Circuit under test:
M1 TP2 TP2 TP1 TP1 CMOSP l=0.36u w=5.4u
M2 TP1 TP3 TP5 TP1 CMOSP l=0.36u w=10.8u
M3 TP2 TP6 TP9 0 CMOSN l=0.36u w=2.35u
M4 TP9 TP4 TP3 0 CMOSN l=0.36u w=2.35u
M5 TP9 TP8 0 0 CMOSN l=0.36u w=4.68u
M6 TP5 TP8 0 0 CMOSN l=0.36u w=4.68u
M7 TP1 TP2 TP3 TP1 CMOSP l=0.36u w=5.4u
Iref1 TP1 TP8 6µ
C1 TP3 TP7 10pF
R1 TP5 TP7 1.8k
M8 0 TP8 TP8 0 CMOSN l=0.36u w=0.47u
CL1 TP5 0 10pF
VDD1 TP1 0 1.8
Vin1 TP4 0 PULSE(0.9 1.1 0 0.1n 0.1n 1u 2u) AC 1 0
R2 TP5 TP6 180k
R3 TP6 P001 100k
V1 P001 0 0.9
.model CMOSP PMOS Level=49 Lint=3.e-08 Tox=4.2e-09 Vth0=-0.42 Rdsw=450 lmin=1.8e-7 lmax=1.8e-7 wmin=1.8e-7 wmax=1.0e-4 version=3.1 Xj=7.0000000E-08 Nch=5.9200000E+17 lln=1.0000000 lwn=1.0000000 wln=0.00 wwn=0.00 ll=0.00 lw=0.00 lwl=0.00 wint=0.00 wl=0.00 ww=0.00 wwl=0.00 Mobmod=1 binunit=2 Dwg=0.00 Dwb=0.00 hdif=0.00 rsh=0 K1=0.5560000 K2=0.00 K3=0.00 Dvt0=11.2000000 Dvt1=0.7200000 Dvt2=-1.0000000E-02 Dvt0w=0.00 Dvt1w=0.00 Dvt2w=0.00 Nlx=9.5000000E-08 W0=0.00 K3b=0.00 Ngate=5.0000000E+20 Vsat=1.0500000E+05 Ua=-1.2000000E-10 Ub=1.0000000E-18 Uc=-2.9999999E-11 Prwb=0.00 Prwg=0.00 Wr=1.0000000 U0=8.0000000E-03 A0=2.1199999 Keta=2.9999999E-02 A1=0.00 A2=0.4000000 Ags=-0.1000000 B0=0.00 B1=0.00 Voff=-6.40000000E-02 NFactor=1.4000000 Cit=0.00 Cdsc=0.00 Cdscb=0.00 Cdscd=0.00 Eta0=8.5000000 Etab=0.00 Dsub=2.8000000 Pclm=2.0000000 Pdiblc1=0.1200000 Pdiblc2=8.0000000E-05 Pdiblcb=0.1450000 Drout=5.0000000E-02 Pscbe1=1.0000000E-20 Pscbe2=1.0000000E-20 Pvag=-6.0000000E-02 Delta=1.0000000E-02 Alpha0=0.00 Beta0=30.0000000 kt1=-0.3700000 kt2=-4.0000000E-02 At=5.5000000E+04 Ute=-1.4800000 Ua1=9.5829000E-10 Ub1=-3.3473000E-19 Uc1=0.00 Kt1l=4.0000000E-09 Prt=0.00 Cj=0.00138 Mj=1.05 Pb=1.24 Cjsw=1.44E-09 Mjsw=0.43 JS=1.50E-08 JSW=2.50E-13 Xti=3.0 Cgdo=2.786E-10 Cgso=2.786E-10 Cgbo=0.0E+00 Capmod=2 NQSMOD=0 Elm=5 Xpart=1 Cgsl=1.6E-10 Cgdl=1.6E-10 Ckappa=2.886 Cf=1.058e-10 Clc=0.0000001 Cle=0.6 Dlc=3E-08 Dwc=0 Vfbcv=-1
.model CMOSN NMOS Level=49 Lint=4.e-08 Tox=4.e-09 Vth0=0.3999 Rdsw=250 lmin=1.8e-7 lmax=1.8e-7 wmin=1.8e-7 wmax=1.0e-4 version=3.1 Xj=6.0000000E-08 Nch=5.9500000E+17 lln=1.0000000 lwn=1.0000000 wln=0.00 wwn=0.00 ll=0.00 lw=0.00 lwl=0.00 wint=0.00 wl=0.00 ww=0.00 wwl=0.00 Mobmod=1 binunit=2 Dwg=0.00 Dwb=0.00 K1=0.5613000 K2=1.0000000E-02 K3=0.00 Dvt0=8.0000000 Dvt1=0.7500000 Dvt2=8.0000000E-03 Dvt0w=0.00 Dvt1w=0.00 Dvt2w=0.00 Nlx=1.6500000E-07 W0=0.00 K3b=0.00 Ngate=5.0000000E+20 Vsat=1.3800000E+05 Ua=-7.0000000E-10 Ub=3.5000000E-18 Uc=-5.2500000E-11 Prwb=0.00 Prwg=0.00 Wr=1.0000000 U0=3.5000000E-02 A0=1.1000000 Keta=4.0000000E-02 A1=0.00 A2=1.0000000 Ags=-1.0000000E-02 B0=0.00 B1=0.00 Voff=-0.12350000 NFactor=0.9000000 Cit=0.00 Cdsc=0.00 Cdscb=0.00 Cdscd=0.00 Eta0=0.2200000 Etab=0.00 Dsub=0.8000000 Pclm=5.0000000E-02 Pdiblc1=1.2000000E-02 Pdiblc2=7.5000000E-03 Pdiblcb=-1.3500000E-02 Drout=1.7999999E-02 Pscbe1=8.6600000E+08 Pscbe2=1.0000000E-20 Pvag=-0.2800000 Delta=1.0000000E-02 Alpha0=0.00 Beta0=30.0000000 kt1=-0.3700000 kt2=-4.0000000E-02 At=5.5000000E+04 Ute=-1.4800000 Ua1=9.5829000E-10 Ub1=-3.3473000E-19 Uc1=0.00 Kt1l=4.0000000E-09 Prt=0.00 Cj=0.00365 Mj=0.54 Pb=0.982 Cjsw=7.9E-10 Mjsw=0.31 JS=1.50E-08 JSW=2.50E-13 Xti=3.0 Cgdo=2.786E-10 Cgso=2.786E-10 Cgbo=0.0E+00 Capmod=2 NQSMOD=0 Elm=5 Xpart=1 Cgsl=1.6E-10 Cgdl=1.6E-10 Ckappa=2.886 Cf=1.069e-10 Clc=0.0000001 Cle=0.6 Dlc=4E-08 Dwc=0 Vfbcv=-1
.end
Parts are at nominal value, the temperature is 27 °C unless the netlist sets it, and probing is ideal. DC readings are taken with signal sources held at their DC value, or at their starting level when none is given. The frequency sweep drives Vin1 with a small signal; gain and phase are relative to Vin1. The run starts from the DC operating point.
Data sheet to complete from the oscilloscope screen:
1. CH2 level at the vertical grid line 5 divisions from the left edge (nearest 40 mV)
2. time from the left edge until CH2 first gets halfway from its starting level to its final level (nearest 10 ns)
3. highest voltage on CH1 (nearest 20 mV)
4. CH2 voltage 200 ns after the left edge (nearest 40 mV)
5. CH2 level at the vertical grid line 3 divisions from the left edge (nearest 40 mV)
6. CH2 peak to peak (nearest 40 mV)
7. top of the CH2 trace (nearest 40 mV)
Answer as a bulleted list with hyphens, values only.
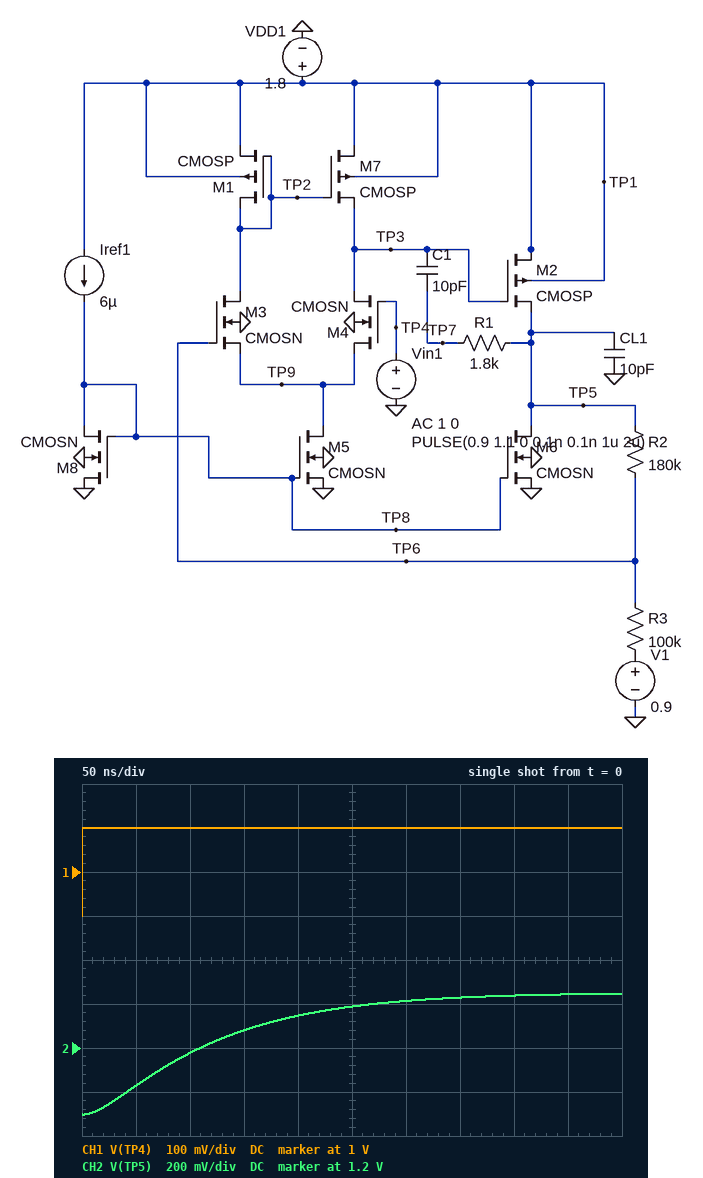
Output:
- 1.40 V
- 100 ns
- 1.10 V
- 1.36 V
- 1.28 V
- 560 mV
- 1.44 V
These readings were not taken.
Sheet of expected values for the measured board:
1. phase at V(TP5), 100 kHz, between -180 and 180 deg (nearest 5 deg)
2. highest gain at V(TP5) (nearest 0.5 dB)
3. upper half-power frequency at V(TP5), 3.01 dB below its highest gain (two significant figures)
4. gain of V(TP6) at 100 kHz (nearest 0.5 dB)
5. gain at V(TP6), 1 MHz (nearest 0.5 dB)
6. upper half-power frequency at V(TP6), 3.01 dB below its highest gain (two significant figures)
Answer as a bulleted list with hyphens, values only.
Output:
- -5 deg
- 9.0 dB
- 1.6 MHz
- 0 dB
- -1.5 dB
- 1.6 MHz
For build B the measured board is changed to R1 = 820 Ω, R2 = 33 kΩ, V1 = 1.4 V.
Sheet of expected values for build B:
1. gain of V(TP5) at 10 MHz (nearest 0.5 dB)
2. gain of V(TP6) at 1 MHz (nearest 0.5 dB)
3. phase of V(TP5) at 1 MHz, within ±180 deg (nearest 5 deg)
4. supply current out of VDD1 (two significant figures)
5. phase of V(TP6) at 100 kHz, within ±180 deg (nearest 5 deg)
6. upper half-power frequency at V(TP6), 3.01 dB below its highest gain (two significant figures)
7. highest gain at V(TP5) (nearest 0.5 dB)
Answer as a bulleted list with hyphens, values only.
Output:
- -8.5 dB
- 0 dB
- -20 deg
- 110 µA
- 0 deg
- 5.2 MHz
- 2.5 dB
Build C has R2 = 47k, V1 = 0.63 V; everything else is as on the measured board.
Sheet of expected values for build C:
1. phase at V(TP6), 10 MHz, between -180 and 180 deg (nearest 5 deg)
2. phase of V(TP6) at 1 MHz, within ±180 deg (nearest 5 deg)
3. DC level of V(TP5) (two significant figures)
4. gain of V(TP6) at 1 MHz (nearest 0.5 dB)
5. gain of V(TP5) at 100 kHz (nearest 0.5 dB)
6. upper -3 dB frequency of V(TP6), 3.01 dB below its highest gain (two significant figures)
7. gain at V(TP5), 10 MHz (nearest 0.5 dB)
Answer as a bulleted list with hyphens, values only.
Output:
- -145 deg
- -25 deg
- 1.0 V
- -0.5 dB
- 3.5 dB
- 3.4 MHz
- -11.0 dB
